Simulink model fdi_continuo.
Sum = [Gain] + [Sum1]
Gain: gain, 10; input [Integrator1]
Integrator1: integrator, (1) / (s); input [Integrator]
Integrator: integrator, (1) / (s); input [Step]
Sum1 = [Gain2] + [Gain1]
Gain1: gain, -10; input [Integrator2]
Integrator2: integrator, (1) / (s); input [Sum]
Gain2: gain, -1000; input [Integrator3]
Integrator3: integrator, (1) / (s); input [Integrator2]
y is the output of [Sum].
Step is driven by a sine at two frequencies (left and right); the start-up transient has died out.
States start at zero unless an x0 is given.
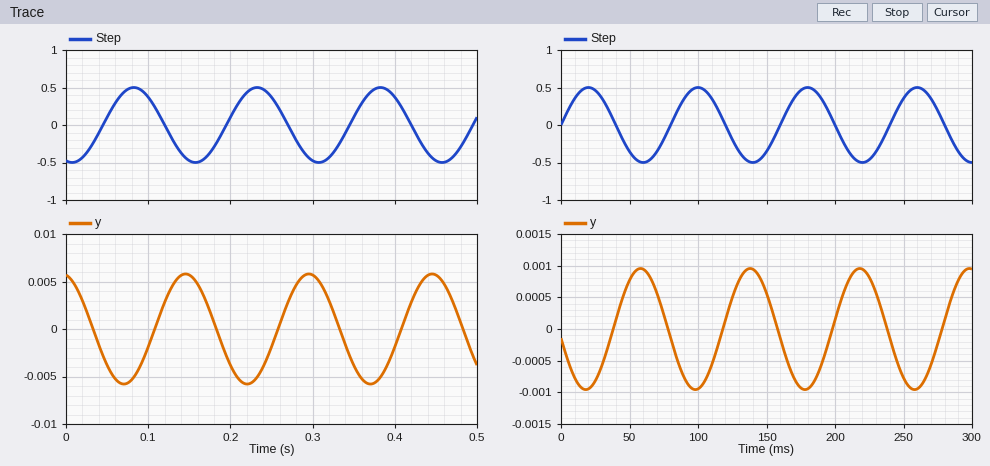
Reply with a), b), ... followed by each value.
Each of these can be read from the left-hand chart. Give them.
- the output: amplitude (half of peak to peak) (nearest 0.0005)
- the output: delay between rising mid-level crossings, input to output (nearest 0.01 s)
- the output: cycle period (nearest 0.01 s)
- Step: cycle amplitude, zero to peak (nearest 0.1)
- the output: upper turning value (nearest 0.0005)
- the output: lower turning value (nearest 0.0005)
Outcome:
a) 0.0060
b) 0.06 s
c) 0.15 s
d) 0.5
e) 0.0060
f) -0.0060
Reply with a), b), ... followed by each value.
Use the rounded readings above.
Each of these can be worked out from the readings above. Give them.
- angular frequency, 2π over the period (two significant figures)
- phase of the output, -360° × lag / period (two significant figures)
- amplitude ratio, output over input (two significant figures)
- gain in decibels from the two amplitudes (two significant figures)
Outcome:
a) 42 rad/s
b) -140°
c) 0.012
d) -38 dB
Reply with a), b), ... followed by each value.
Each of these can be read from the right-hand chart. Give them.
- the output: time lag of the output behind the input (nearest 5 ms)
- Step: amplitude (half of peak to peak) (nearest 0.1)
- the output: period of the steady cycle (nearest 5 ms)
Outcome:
a) 40 ms
b) 0.5
c) 80 ms
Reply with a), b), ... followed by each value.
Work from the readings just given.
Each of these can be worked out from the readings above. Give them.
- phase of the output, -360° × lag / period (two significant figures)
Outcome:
a) -180°
